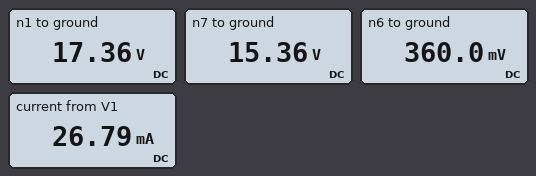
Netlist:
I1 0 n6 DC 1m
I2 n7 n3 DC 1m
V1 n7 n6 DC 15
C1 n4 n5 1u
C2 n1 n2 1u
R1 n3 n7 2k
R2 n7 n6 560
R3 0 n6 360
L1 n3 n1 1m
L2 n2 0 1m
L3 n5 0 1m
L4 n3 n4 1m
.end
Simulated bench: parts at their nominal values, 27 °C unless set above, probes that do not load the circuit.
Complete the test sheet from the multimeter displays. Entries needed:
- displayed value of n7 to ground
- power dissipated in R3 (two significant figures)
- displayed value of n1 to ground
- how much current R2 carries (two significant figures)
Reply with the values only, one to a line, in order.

15.36 V
360 µW
17.36 V
27 mA
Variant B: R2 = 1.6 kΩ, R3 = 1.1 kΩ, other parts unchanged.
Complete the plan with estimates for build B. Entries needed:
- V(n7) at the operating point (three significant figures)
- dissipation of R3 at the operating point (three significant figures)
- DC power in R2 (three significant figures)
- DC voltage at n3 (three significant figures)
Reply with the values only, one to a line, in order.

16.1 V
1.10 mW
141 mW
18.1 V
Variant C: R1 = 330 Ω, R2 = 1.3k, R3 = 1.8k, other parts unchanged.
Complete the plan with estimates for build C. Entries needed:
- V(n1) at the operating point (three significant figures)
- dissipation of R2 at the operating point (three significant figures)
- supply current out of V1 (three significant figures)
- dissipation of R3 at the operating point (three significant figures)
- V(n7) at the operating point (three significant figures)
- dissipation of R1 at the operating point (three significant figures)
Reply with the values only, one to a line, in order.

17.1 V
173 mW
11.5 mA
1.80 mW
16.8 V
330 µW
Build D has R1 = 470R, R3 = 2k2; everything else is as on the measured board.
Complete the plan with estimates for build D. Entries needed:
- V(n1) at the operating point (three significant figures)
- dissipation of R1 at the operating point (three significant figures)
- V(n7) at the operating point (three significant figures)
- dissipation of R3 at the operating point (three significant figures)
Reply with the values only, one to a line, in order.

17.7 V
470 µW
17.2 V
2.20 mW
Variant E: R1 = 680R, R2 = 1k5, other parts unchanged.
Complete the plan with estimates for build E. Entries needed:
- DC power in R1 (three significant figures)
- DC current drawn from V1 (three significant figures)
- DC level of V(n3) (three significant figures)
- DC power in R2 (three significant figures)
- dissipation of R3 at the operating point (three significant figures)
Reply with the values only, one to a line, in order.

680 µW
10.0 mA
16.0 V
150 mW
360 µW
